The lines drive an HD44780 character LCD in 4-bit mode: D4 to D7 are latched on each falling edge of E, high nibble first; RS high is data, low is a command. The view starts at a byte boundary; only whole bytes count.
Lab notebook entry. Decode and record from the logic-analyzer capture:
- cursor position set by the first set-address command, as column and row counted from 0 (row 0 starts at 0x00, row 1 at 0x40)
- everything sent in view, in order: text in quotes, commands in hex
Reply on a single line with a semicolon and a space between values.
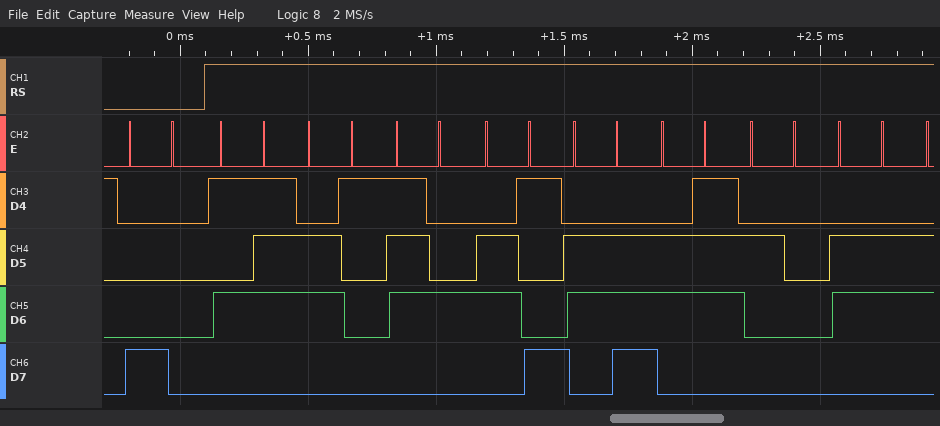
column 0, row 0; 0x80 "Wating f"
